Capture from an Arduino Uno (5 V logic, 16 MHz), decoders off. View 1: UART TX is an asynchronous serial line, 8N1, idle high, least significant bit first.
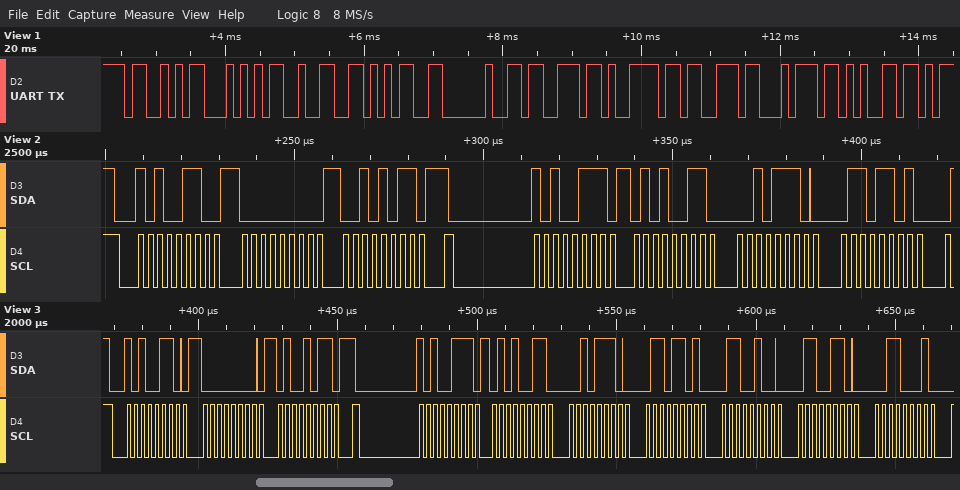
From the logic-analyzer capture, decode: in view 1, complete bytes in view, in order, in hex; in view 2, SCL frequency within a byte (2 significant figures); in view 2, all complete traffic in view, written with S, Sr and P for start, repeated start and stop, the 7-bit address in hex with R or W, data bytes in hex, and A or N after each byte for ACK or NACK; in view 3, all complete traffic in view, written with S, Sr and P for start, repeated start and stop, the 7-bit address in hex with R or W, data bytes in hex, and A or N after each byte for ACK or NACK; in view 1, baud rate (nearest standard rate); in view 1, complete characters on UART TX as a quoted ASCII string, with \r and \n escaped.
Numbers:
0x53 0x54 0x32 0x35 0x20 0x73 0x79 0x73 0x74 0x65
400 kHz
S 53W A 00 A 2B A Sr 53R A 53 A 2E A 6D A
S 53W A 00 A 4B A Sr 53R A 53 A 2E A 6D A 64 A 66 A 31 A
9600 baud
"ST25 syste"
